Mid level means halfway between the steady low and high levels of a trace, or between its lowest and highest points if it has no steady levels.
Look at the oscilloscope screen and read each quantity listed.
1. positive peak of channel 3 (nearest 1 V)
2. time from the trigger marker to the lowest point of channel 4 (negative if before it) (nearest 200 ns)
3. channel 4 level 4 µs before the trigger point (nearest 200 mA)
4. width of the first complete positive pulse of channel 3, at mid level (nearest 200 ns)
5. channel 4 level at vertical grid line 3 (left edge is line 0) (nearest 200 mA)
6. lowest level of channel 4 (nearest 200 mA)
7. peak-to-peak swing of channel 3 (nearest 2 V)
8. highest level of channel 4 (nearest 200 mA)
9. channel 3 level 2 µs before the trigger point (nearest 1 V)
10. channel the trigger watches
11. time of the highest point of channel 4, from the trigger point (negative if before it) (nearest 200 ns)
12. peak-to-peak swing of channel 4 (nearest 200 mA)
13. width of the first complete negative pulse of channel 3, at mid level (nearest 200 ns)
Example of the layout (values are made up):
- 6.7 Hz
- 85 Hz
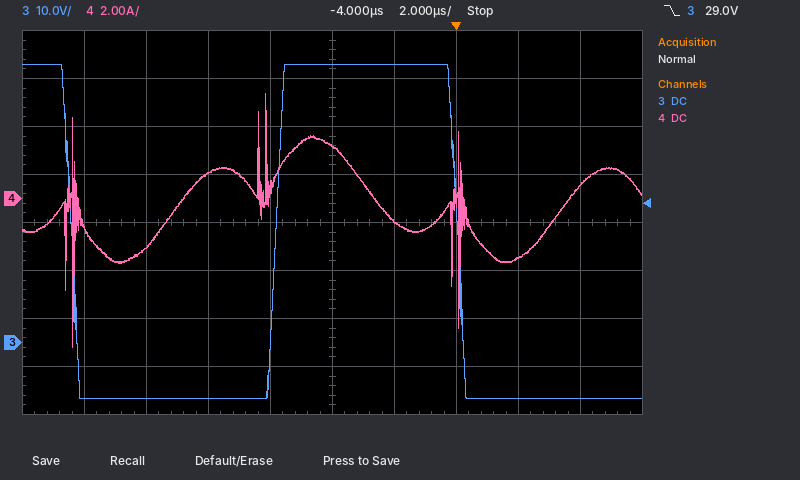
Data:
- 58 V
- -12.4 µs
- 2.2 A
- 5.8 µs
- 1.0 A
- -6.2 A
- 70 V
- 4.4 A
- 58 V
- channel 3
- -6.2 µs
- 10.6 A
- 6.6 µs
